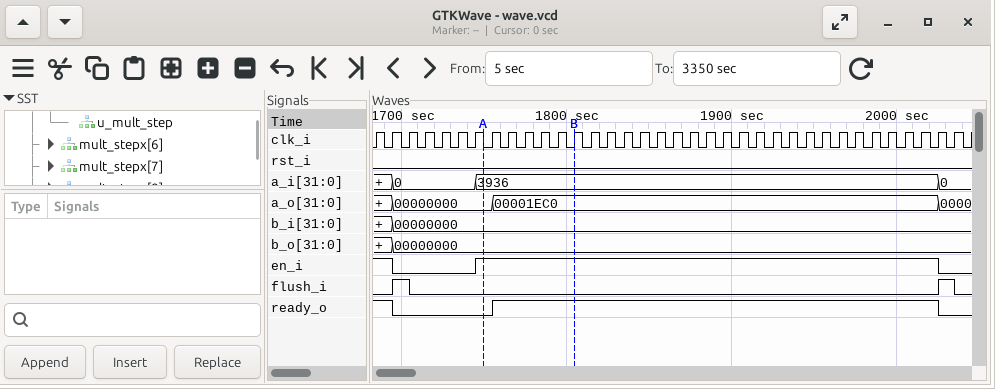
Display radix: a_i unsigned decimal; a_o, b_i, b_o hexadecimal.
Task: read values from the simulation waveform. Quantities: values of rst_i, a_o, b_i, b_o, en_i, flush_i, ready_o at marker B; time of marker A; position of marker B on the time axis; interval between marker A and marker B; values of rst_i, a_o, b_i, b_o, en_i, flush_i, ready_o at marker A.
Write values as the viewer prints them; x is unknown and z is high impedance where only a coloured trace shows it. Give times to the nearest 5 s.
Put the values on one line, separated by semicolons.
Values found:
rst_i=0, a_o=00001EC0, b_i=00000000, b_o=00000000, en_i=1, flush_i=0, ready_o=1; 1750 s; 1805 s; 55 s; rst_i=0, a_o=00000000, b_i=00000000, b_o=00000000, en_i=1, flush_i=0, ready_o=0
